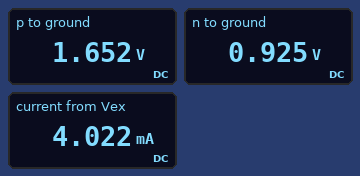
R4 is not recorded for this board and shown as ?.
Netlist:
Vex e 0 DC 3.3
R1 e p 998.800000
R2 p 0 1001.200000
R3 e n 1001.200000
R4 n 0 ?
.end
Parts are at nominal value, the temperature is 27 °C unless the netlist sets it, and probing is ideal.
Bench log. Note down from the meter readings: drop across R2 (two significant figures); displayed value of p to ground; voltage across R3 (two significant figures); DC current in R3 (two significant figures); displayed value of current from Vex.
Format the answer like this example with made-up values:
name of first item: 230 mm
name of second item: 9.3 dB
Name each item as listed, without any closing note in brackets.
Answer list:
drop across R2: 1.7 V
displayed value of p to ground: 1.652 V
voltage across R3: 2.4 V
DC current in R3: 2.4 mA
displayed value of current from Vex: 4.022 mA
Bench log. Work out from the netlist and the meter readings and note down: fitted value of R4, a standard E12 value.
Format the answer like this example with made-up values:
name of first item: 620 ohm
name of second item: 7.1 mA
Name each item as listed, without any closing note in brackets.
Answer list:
fitted value of R4, a standard E12 value: 390 Ω
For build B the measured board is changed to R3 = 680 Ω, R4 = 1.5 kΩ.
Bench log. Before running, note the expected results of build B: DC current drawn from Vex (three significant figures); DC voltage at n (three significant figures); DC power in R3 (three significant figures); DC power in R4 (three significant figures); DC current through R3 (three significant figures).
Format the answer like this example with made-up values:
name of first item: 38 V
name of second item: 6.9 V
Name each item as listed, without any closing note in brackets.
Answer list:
DC current drawn from Vex: 3.16 mA
DC voltage at n: 2.27 V
DC power in R3: 1.56 mW
DC power in R4: 3.44 mW
DC current through R3: 1.51 mA
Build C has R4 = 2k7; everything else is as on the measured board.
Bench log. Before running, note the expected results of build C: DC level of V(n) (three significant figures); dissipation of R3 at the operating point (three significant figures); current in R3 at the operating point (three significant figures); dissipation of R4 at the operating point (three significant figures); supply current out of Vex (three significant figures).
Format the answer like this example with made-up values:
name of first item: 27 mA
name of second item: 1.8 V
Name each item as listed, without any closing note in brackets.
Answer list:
DC level of V(n): 2.41 V
dissipation of R3 at the operating point: 796 µW
current in R3 at the operating point: 892 µA
dissipation of R4 at the operating point: 2.15 mW
supply current out of Vex: 2.54 mA
